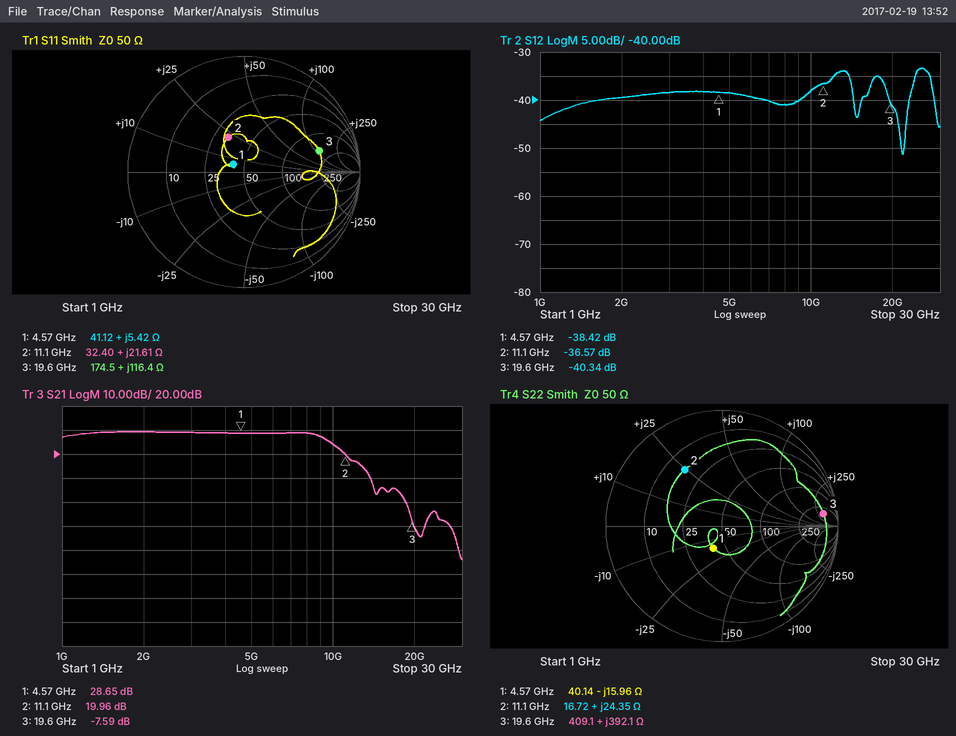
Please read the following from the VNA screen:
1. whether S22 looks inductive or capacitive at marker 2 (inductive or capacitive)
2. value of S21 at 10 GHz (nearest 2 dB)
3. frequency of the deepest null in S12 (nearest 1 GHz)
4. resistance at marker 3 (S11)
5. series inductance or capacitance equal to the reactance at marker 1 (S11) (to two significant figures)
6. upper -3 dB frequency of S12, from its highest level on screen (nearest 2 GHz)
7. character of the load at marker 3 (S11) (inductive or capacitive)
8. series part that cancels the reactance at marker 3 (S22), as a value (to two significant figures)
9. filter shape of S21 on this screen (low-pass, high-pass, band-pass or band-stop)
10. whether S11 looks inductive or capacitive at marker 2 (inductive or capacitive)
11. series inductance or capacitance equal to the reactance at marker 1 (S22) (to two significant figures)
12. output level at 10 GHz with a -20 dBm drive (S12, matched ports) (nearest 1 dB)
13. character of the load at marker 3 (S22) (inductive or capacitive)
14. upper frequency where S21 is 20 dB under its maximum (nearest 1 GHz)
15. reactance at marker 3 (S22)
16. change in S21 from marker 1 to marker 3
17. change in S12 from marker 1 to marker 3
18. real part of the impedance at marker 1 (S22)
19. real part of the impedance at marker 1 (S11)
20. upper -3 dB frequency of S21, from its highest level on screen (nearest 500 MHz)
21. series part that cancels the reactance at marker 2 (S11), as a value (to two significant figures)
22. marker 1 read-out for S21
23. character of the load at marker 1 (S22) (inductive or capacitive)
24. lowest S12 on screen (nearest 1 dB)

inductive
24 dB
22 GHz
174.5 Ω
190 pH
28 GHz
inductive
21 fF
low-pass
inductive
2.2 pF
-58 dBm
inductive
14 GHz
+392.1 Ω
-36.24 dB
-1.92 dB
40.14 Ω
41.12 Ω
9.5 GHz
660 fF
28.65 dB
capacitive
-51 dB
